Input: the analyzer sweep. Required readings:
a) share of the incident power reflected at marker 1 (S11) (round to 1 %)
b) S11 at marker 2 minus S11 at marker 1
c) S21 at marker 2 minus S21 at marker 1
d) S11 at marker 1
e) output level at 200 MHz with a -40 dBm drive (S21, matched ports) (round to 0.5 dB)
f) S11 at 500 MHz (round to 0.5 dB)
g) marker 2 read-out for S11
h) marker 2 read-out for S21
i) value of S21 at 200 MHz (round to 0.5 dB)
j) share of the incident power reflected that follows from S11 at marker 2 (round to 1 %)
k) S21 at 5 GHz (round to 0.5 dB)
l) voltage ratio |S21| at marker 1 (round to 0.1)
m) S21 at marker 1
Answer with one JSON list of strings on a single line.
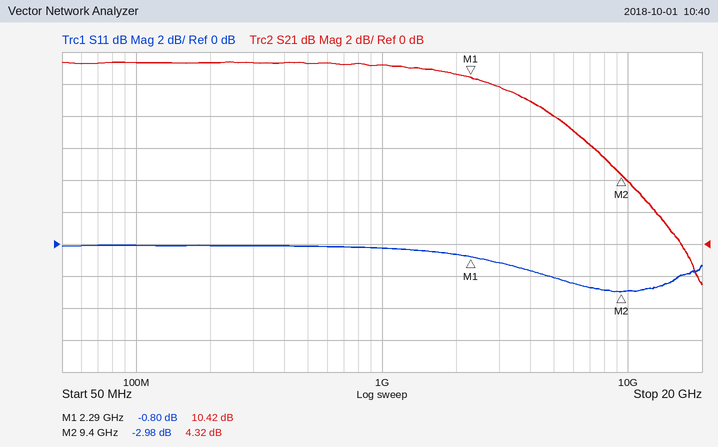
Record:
["83 %", "-2.18 dB", "-6.10 dB", "-0.80 dB", "-28.5 dBm", "0.0 dB", "-2.98 dB", "4.32 dB", "11.5 dB", "50 %", "8.0 dB", "3.3", "10.42 dB"]
